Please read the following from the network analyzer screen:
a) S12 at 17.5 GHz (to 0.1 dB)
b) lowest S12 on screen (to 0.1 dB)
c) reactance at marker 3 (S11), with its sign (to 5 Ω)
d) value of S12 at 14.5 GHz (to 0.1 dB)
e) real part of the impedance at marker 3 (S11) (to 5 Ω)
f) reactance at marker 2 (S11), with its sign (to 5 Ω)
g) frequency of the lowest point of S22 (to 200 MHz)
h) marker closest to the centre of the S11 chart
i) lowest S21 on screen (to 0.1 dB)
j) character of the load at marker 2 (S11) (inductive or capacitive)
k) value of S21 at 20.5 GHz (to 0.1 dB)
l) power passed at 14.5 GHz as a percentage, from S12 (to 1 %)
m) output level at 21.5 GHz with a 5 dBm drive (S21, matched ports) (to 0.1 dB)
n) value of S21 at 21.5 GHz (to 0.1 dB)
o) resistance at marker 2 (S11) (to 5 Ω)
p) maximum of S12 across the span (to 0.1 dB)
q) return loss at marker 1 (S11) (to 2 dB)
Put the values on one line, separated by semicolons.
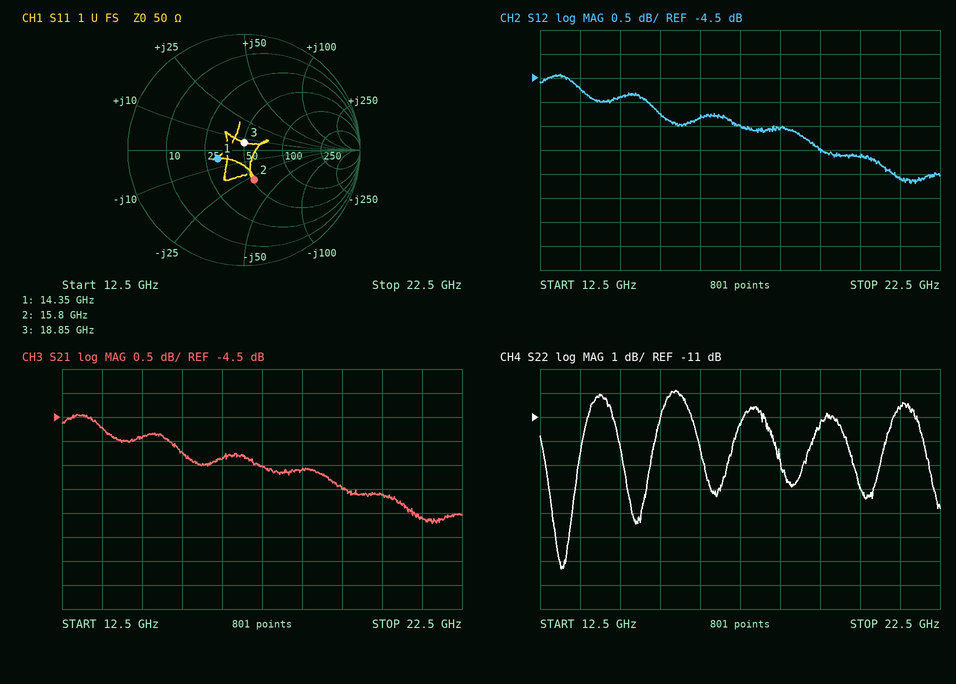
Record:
-5.5 dB; -6.7 dB; +5 Ω; -4.9 dB; 50 Ω; -30 Ω; 13.0 GHz; marker 3; -6.7 dB; capacitive; -6.1 dB; 32 %; -1.6 dBm; -6.6 dB; 50 Ω; -4.4 dB; 12 dB
